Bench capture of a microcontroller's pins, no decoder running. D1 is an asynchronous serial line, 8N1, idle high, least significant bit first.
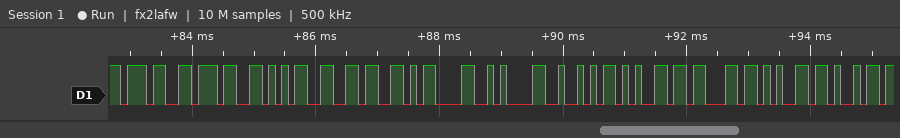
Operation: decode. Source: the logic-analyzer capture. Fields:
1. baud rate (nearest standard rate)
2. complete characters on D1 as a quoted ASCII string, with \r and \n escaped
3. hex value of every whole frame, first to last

9600 baud
"7756\r\nRecei"
37 37 35 36 0D 0A 52 65 63 65 69
